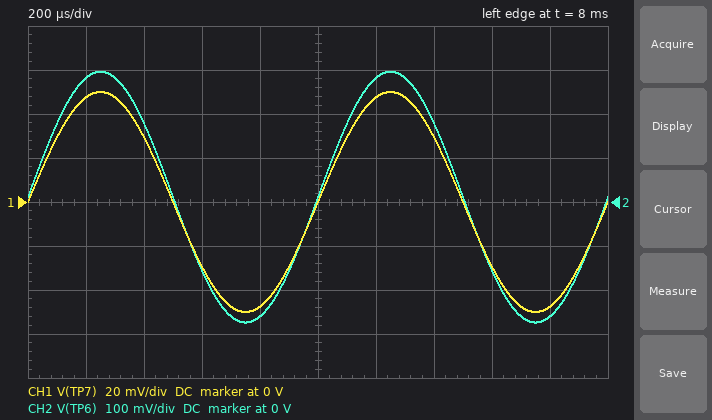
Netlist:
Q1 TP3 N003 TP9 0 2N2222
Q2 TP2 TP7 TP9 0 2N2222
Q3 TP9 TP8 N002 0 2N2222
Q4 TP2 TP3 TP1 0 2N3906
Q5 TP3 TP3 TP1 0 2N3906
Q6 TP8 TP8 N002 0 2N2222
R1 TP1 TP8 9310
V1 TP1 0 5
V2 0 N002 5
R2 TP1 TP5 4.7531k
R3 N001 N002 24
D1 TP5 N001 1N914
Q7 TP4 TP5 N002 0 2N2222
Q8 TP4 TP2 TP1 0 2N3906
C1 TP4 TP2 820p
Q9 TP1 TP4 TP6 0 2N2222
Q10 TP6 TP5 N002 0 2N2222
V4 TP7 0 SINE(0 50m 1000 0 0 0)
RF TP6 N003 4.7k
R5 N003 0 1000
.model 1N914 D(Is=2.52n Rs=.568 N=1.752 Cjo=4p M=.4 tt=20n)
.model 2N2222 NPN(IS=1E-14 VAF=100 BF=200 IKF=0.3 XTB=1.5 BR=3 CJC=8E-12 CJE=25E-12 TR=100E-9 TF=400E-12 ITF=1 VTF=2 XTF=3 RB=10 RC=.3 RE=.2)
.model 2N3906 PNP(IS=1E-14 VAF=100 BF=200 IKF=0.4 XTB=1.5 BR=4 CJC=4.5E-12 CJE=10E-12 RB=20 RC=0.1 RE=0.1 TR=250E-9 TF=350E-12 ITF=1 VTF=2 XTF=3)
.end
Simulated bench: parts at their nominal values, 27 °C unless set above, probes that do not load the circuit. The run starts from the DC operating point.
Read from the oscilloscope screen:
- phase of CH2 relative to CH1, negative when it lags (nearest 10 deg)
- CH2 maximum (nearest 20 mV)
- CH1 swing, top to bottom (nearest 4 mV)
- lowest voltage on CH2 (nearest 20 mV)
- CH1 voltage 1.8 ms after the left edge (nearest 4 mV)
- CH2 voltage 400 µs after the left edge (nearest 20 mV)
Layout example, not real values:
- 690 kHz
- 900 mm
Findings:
- 0 deg
- 300 mV
- 100 mV
- -280 mV
- -48 mV
- 180 mV
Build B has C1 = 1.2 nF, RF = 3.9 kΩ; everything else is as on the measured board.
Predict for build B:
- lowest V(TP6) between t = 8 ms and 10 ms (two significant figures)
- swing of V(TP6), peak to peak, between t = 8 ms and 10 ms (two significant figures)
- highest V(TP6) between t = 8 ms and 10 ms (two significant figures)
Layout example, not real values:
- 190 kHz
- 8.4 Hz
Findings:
- -240 mV
- 490 mV
- 250 mV
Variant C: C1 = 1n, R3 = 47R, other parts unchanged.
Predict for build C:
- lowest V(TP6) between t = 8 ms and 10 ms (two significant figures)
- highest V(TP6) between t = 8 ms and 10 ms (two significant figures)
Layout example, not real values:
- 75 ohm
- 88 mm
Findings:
- -280 mV
- 290 mV
